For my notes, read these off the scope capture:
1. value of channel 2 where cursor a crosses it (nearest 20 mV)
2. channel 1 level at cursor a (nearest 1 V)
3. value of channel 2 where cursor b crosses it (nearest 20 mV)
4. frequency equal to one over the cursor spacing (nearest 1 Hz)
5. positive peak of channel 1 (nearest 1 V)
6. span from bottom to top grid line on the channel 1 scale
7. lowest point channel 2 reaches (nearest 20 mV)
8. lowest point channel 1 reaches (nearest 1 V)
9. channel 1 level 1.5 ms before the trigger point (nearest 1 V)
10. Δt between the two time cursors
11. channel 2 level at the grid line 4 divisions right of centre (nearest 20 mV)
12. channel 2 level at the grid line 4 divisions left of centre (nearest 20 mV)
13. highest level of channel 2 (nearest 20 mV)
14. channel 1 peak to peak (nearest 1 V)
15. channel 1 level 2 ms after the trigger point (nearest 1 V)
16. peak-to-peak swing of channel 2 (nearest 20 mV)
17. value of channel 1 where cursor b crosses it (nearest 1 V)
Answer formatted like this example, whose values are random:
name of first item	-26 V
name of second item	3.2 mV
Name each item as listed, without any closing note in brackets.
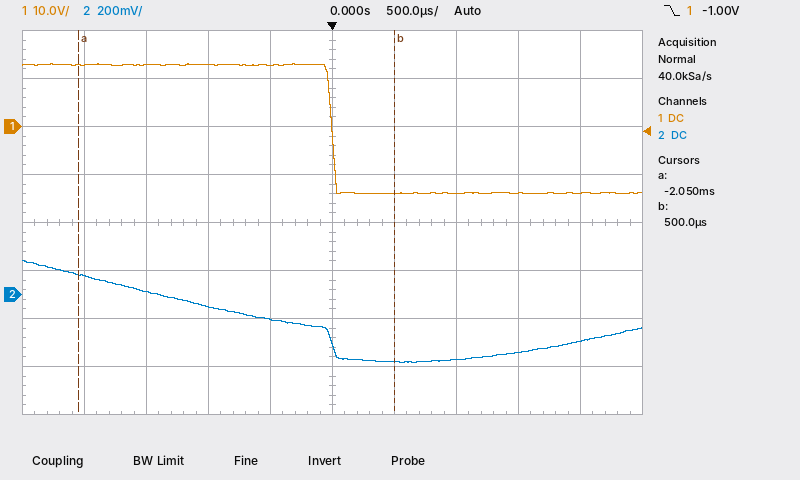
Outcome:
value of channel 2 where cursor a crosses it	80 mV
channel 1 level at cursor a	13 V
value of channel 2 where cursor b crosses it	-280 mV
frequency equal to one over the cursor spacing	392 Hz
positive peak of channel 1	13 V
span from bottom to top grid line on the channel 1 scale	80 V
lowest point channel 2 reaches	-280 mV
lowest point channel 1 reaches	-14 V
channel 1 level 1.5 ms before the trigger point	13 V
Δt between the two time cursors	2.55 ms
channel 2 level at the grid line 4 divisions right of centre	-200 mV
channel 2 level at the grid line 4 divisions left of centre	80 mV
highest level of channel 2	140 mV
channel 1 peak to peak	27 V
channel 1 level 2 ms after the trigger point	-14 V
peak-to-peak swing of channel 2	420 mV
value of channel 1 where cursor b crosses it	-14 V
